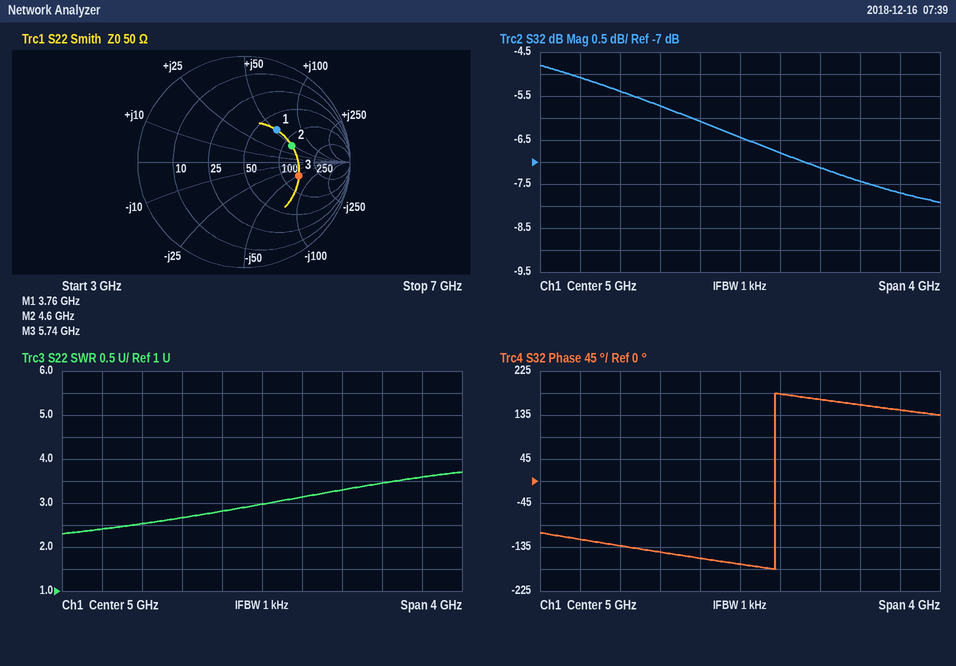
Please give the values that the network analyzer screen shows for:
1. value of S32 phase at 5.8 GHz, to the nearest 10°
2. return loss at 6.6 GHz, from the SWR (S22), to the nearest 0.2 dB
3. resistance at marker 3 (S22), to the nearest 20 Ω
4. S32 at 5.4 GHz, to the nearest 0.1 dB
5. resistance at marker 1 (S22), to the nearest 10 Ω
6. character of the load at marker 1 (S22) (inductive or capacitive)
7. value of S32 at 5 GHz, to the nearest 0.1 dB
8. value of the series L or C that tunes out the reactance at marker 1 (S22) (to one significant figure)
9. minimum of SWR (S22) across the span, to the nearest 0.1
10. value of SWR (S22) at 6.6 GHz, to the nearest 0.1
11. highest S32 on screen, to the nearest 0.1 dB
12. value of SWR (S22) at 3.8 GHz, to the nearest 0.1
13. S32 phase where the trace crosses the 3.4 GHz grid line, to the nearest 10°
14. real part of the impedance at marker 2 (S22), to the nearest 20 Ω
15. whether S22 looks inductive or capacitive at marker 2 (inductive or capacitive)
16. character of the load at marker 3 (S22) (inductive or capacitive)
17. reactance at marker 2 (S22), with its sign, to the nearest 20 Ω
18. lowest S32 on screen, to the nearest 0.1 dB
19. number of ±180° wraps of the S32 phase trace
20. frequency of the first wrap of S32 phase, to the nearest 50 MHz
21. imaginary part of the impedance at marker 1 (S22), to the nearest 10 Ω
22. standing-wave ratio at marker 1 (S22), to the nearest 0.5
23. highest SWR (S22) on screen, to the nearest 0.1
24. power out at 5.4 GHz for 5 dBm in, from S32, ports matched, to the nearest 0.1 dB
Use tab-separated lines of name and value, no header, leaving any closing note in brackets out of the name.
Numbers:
value of S32 phase at 5.8 GHz, to the nearest 10°	170°
return loss at 6.6 GHz, from the SWR (S22), to the nearest 0.2 dB	5.0 dB
resistance at marker 3 (S22), to the nearest 20 Ω	140 Ω
S32 at 5.4 GHz, to the nearest 0.1 dB	-6.8 dB
resistance at marker 1 (S22), to the nearest 10 Ω	70 Ω
character of the load at marker 1 (S22)	inductive
value of S32 at 5 GHz, to the nearest 0.1 dB	-6.4 dB
value of the series L or C that tunes out the reactance at marker 1 (S22)	800 fF
minimum of SWR (S22) across the span, to the nearest 0.1	2.3
value of SWR (S22) at 6.6 GHz, to the nearest 0.1	3.6
highest S32 on screen, to the nearest 0.1 dB	-4.8 dB
value of SWR (S22) at 3.8 GHz, to the nearest 0.1	2.5
S32 phase where the trace crosses the 3.4 GHz grid line, to the nearest 10°	-120°
real part of the impedance at marker 2 (S22), to the nearest 20 Ω	120 Ω
whether S22 looks inductive or capacitive at marker 2	inductive
character of the load at marker 3 (S22)	capacitive
reactance at marker 2 (S22), with its sign, to the nearest 20 Ω	+40 Ω
lowest S32 on screen, to the nearest 0.1 dB	-7.9 dB
number of ±180° wraps of the S32 phase trace	1
frequency of the first wrap of S32 phase, to the nearest 50 MHz	5.35 GHz
imaginary part of the impedance at marker 1 (S22), to the nearest 10 Ω	+50 Ω
standing-wave ratio at marker 1 (S22), to the nearest 0.5	2.5
highest SWR (S22) on screen, to the nearest 0.1	3.7
power out at 5.4 GHz for 5 dBm in, from S32, ports matched, to the nearest 0.1 dB	-1.8 dBm
